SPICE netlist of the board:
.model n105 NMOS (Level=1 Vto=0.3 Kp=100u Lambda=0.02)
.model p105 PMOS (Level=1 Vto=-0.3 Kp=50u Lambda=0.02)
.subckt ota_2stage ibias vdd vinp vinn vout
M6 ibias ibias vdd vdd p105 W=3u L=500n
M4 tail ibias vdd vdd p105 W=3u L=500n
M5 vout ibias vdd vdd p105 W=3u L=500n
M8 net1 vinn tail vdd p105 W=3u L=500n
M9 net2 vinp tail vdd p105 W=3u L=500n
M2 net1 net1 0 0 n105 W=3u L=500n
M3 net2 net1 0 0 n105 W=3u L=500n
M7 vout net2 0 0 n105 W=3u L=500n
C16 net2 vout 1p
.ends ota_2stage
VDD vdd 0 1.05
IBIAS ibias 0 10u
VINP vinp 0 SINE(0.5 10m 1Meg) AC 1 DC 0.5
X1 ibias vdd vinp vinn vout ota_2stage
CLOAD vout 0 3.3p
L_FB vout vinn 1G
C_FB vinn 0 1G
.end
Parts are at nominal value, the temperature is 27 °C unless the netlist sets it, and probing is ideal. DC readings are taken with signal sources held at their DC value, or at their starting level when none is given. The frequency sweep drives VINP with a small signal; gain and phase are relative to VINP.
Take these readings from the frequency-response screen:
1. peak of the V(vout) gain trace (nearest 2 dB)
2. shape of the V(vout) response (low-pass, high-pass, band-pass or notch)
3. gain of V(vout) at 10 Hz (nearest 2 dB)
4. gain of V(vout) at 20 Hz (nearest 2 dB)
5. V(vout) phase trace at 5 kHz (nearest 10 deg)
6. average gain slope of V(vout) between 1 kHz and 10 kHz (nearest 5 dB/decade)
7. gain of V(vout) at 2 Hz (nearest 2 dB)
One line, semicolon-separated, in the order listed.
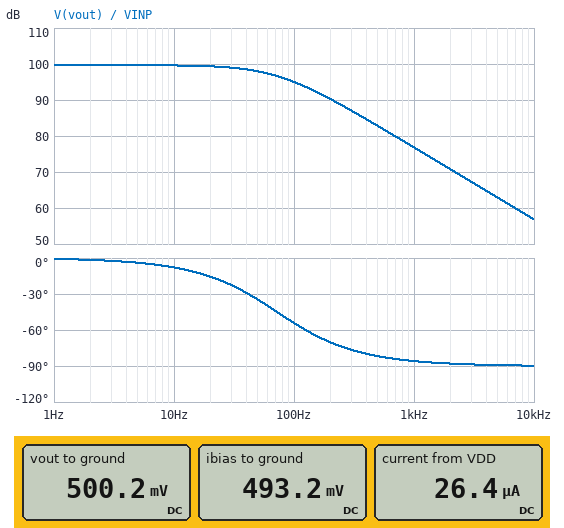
100 dB; low-pass; 100 dB; 100 dB; -90 deg; -20 dB/decade; 100 dB
